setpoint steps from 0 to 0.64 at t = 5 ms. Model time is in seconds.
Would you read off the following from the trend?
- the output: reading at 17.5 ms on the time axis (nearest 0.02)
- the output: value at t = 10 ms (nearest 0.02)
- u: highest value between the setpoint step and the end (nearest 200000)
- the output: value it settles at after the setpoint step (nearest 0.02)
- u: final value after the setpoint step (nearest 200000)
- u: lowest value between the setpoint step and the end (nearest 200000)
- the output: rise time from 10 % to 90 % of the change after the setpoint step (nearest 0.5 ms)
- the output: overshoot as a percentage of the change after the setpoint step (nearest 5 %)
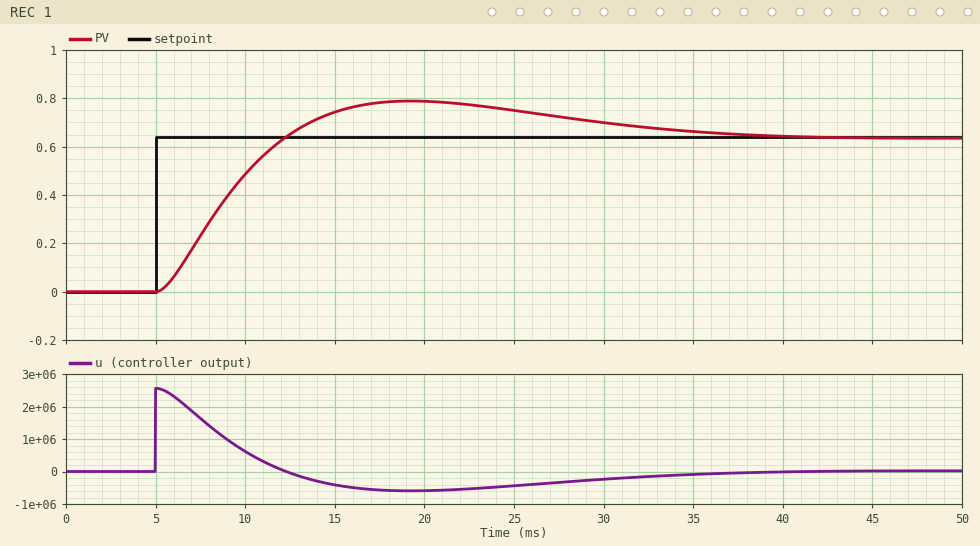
0.78
0.48
2600000
0.64
0
-600000
5.0 ms
25 %
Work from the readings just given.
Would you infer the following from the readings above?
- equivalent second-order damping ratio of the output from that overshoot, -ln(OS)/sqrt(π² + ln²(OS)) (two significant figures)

0.40
